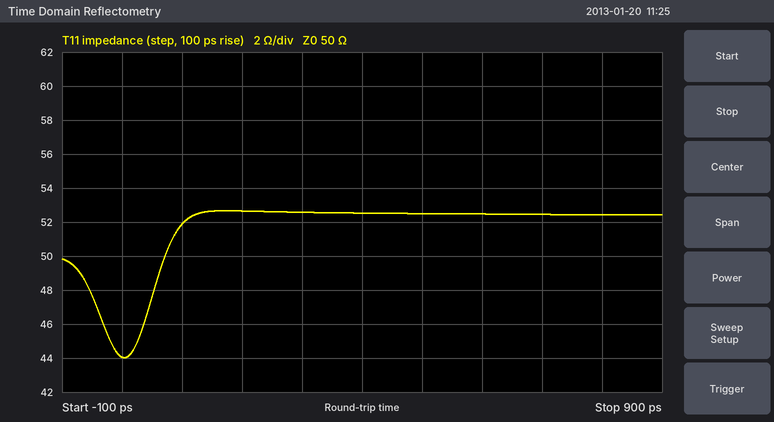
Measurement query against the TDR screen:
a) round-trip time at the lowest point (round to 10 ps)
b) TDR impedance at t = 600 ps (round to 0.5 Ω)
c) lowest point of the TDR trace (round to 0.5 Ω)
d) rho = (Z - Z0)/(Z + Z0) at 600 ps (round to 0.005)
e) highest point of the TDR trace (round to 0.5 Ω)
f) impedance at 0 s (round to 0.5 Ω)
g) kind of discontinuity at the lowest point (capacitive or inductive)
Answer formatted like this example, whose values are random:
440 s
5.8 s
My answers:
0 ps
52.5 Ω
44.0 Ω
+0.025
52.5 Ω
44.0 Ω
capacitive
